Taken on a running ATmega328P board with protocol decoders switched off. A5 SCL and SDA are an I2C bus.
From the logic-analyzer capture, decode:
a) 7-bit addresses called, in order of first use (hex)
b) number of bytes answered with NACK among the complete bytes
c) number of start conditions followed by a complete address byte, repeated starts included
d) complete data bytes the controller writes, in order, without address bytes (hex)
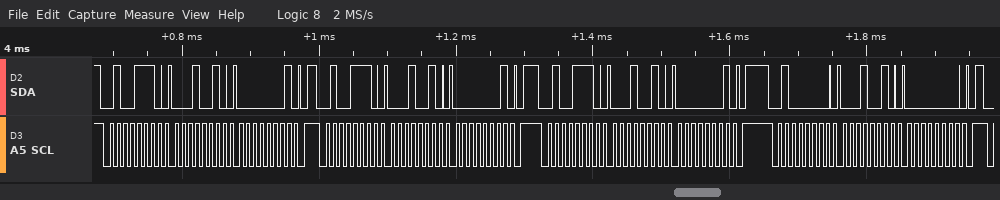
0x27 0x20
0
4
12 01 12 01 12 01 12 00
